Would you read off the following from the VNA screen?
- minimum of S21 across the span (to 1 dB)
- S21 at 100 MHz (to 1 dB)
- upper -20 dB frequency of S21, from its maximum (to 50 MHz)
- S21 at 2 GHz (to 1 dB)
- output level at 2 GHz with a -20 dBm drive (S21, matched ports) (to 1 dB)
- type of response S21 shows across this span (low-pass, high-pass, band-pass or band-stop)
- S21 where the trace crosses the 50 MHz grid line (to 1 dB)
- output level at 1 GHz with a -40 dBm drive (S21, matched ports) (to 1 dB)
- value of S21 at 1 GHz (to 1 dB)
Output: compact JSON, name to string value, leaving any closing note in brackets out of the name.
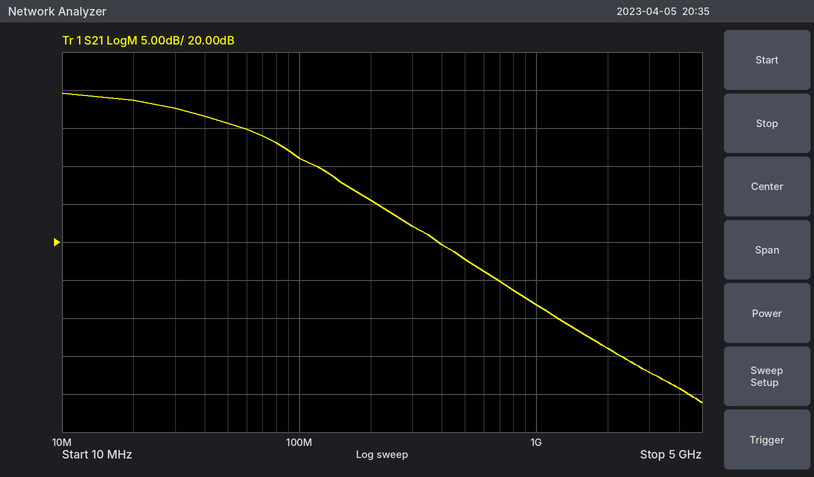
{"minimum of S21 across the span": "-1 dB", "S21 at 100 MHz": "31 dB", "upper -20 dB frequency of S21, from its maximum": "400 MHz", "S21 at 2 GHz": "6 dB", "output level at 2 GHz with a -20 dBm drive (S21, matched ports)": "-14 dBm", "type of response S21 shows across this span": "low-pass", "S21 where the trace crosses the 50 MHz grid line": "36 dB", "output level at 1 GHz with a -40 dBm drive (S21, matched ports)": "-28 dBm", "value of S21 at 1 GHz": "12 dB"}
